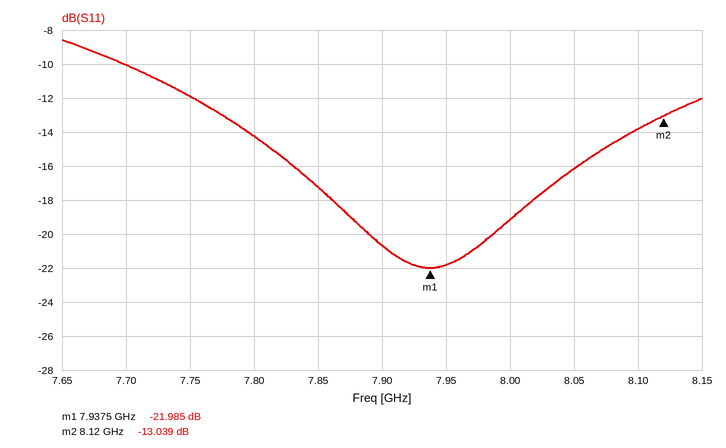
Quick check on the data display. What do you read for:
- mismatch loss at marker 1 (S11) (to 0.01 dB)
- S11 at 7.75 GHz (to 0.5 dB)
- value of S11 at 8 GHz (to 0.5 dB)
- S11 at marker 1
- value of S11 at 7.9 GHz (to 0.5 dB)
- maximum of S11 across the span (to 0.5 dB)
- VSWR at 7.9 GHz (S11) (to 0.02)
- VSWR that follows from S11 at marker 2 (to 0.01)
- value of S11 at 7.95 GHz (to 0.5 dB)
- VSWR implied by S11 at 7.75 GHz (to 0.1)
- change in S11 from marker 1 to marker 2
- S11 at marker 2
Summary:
0.03 dB
-12.0 dB
-19.0 dB
-21.985 dB
-20.5 dB
-8.5 dB
1.20
1.57
-22.0 dB
1.7
8.946 dB
-13.039 dB
